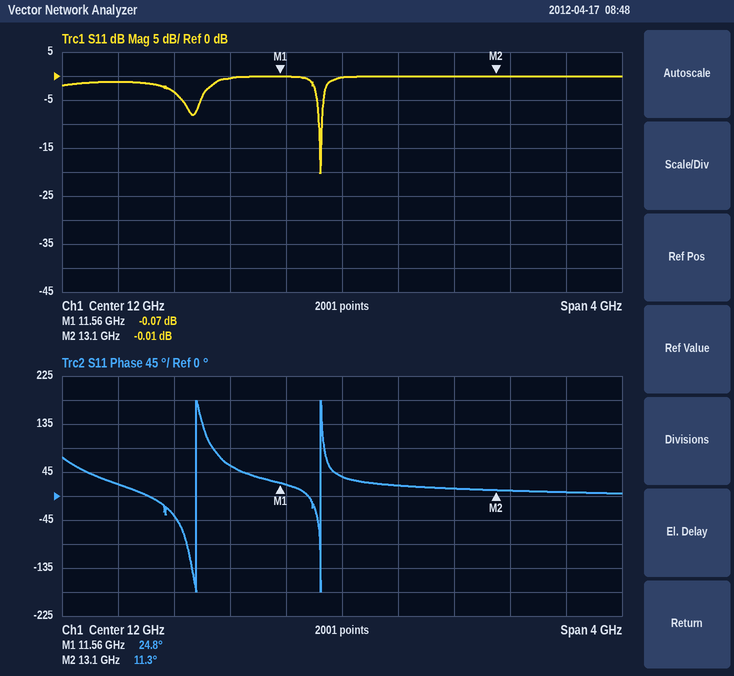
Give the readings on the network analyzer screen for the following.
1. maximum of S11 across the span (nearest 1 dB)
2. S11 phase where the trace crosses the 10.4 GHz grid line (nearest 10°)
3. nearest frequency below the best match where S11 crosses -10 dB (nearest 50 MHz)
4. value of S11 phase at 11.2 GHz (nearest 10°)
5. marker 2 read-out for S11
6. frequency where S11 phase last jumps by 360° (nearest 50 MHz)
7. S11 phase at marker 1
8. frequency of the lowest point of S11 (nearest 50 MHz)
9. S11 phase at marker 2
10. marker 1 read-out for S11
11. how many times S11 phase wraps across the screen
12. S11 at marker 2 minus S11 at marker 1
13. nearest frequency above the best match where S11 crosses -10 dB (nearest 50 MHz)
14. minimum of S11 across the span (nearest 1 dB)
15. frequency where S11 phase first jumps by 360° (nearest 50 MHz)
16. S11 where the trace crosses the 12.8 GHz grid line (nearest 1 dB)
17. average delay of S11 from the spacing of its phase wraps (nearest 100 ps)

0 dB
20°
11.85 GHz
60°
-0.01 dB
11.85 GHz
24.8°
11.85 GHz
11.3°
-0.07 dB
2
0.06 dB
11.85 GHz
-20 dB
10.95 GHz
0 dB
1.1 ns
